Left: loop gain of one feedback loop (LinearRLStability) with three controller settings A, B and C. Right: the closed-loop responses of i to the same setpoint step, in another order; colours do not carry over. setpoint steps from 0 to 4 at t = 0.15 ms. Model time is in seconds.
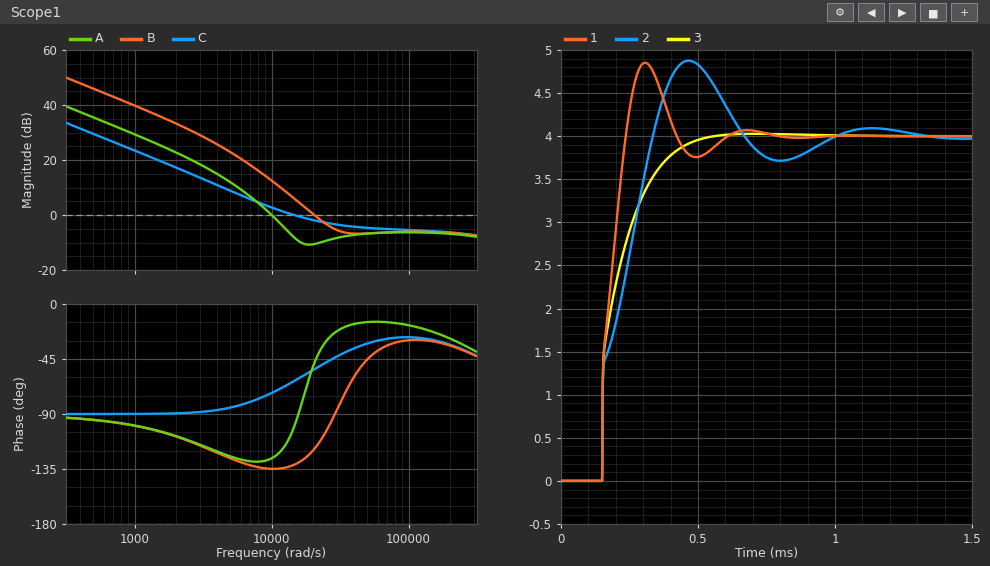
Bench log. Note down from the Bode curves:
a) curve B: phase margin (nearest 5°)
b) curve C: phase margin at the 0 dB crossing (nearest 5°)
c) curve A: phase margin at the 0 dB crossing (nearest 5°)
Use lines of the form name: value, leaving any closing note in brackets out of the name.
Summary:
curve B: phase margin: 60°
curve C: phase margin at the 0 dB crossing: 115°
curve A: phase margin at the 0 dB crossing: 55°
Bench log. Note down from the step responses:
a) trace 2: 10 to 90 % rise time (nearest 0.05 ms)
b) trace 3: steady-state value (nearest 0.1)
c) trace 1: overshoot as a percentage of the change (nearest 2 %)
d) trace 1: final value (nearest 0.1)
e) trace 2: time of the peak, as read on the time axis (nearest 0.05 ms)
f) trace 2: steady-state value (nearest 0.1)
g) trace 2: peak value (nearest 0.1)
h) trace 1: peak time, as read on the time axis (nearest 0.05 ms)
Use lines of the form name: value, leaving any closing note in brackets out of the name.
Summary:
trace 2: 10 to 90 % rise time: 0.15 ms
trace 3: steady-state value: 4.0
trace 1: overshoot as a percentage of the change: 22 %
trace 1: final value: 4.0
trace 2: time of the peak, as read on the time axis: 0.45 ms
trace 2: steady-state value: 4.0
trace 2: peak value: 4.9
trace 1: peak time, as read on the time axis: 0.30 ms
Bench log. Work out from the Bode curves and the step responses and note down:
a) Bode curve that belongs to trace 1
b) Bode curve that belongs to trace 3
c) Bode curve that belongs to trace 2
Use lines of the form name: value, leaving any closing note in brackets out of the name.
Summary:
Bode curve that belongs to trace 1: B
Bode curve that belongs to trace 3: C
Bode curve that belongs to trace 2: A
